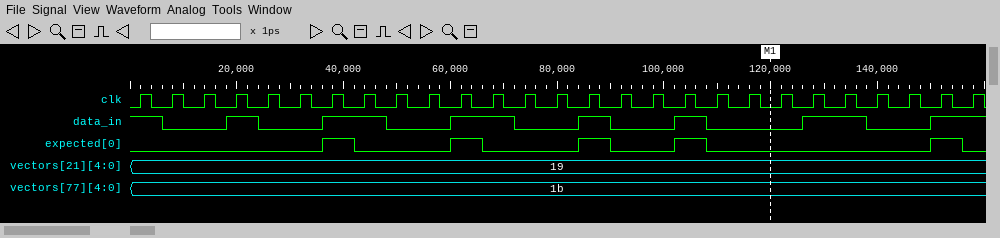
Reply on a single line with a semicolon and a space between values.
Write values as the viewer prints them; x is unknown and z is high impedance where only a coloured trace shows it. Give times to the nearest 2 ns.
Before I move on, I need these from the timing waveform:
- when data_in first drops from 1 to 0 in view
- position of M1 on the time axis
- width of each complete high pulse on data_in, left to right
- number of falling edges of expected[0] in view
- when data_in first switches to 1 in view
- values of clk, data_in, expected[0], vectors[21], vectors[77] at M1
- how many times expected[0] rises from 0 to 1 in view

6 ns; 120 ns; 6 ns, 12 ns, 12 ns, 6 ns, 6 ns, 12 ns; 5; 18 ns; clk=0, data_in=0, expected[0]=0, vectors[21]=19, vectors[77]=1b; 5
